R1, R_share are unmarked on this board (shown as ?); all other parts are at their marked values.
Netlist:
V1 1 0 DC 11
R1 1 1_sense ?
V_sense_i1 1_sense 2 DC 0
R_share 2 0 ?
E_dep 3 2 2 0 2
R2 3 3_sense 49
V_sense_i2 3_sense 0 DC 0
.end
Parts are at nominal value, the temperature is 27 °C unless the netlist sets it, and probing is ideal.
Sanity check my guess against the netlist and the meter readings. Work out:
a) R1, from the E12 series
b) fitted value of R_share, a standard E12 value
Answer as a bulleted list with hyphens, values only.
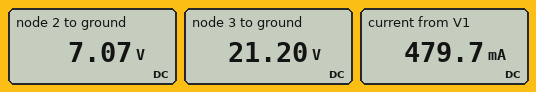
- 8.2 Ω
- 150 Ω
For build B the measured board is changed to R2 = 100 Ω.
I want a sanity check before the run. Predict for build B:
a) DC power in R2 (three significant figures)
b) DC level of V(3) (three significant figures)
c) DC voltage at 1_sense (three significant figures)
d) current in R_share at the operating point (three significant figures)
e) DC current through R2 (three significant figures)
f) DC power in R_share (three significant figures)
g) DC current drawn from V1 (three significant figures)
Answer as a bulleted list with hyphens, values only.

- 6.44 W
- 25.4 V
- 8.46 V
- 56.4 mA
- 254 mA
- 477 mW
- 310 mA
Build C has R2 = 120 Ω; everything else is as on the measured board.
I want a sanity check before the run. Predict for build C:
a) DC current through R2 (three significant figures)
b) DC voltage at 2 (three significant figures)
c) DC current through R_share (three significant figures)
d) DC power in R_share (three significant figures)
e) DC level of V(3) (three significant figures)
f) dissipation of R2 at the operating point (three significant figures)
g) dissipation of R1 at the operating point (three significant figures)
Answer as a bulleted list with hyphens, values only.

- 218 mA
- 8.73 V
- 58.2 mA
- 508 mW
- 26.2 V
- 5.72 W
- 627 mW
